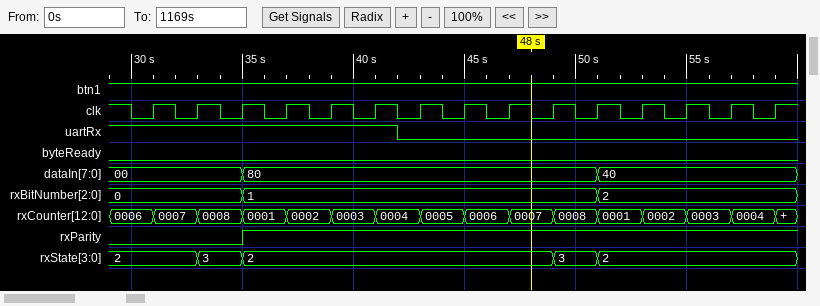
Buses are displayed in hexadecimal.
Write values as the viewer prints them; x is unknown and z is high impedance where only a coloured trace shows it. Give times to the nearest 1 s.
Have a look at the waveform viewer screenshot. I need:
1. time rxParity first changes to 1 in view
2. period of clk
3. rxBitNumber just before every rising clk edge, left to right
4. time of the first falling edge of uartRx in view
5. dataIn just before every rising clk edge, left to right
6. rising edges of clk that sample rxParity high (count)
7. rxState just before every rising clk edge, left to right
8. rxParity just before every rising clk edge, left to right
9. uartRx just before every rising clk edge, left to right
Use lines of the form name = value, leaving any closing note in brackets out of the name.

time rxParity first changes to 1 in view = 35 s
period of clk = 2 s
rxBitNumber just before every rising clk edge, left to right = 0, 0, 0, 1, 1, 1, 1, 1, 1, 1, 1, 2, 2, 2, 2
time of the first falling edge of uartRx in view = 42 s
dataIn just before every rising clk edge, left to right = 00, 00, 00, 80, 80, 80, 80, 80, 80, 80, 80, 40, 40, 40, 40
rising edges of clk that sample rxParity high = 12
rxState just before every rising clk edge, left to right = 2, 2, 3, 2, 2, 2, 2, 2, 2, 2, 3, 2, 2, 2, 2
rxParity just before every rising clk edge, left to right = 0 0 0 1 1 1 1 1 1 1 1 1 1 1 1
uartRx just before every rising clk edge, left to right = 1 1 1 1 1 1 0 0 0 0 0 0 0 0 0
